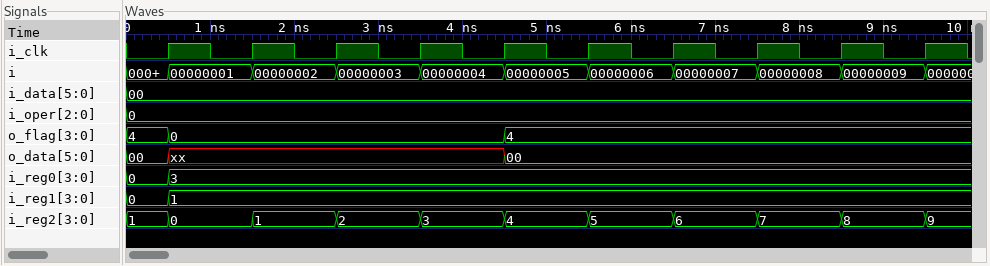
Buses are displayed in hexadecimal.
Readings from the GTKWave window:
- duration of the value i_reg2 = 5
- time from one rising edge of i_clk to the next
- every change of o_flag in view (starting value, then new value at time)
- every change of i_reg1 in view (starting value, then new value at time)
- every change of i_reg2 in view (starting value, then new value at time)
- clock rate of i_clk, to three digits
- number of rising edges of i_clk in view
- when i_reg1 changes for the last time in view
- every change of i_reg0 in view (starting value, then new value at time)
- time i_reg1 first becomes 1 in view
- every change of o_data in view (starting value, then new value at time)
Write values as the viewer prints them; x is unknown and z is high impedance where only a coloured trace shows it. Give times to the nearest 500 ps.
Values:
1000 ps
1000 ps
4, 0 at 500 ps, 4 at 4500 ps
0, 1 at 500 ps
1, 0 at 500 ps, 1 at 1500 ps, 2 at 2500 ps, 3 at 3500 ps, 4 at 4500 ps, 5 at 5500 ps, 6 at 6500 ps, 7 at 7500 ps, 8 at 8500 ps, 9 at 9500 ps
1.00 GHz
10
500 ps
0, 3 at 500 ps
500 ps
00, xx at 500 ps, 00 at 4500 ps
